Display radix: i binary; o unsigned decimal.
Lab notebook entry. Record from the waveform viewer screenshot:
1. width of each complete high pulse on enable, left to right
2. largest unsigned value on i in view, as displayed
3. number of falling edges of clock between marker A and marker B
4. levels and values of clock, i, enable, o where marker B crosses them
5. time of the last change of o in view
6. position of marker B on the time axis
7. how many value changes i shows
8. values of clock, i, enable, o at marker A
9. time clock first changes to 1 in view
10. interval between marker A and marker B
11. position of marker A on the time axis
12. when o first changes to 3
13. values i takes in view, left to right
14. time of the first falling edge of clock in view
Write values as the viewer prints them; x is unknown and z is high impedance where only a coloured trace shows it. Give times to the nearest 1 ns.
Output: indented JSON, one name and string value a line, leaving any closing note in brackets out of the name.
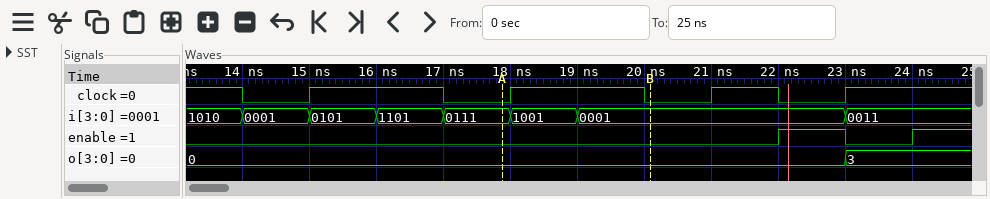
{
  "width of each complete high pulse on enable, left to right": "1 ns",
  "largest unsigned value on i in view, as displayed": "1101",
  "number of falling edges of clock between marker A and marker B": "1",
  "levels and values of clock, i, enable, o where marker B crosses them": "clock=0, i=0001, enable=0, o=0",
  "time of the last change of o in view": "23 ns",
  "position of marker B on the time axis": "20 ns",
  "how many value changes i shows": "7",
  "values of clock, i, enable, o at marker A": "clock=0, i=0111, enable=0, o=0",
  "time clock first changes to 1 in view": "15 ns",
  "interval between marker A and marker B": "2 ns",
  "position of marker A on the time axis": "18 ns",
  "when o first changes to 3": "23 ns",
  "values i takes in view, left to right": "1010, 0001, 0101, 1101, 0111, 1001, 0001, 0011",
  "time of the first falling edge of clock in view": "14 ns"
}
